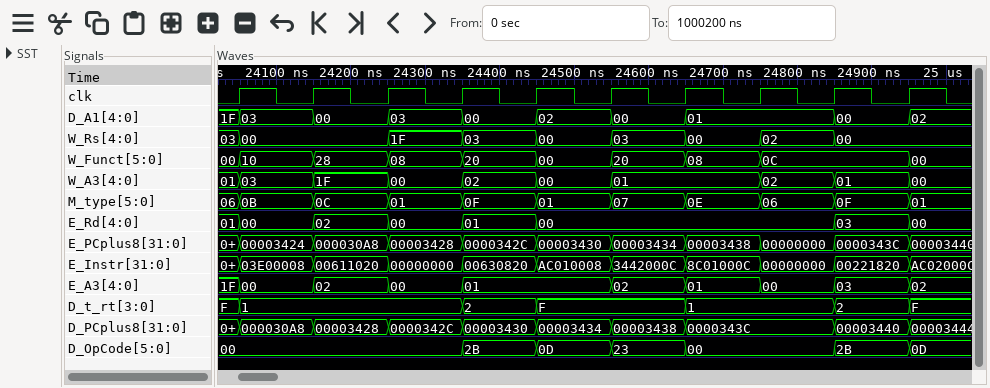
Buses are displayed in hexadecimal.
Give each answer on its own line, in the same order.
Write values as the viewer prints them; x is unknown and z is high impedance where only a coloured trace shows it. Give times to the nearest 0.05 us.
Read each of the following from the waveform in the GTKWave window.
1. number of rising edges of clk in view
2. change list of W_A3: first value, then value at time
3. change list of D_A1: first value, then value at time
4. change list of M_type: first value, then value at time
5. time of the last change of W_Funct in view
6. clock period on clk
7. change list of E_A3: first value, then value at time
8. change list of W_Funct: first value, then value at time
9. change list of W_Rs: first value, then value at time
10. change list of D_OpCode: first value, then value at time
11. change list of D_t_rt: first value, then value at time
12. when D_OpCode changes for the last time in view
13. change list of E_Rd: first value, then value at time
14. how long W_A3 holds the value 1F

10
01, 03 at 24.05 us, 1F at 24.15 us, 00 at 24.25 us, 02 at 24.35 us, 00 at 24.45 us, 01 at 24.55 us, 02 at 24.75 us, 01 at 24.85 us, 00 at 24.95 us
1F, 03 at 24.05 us, 00 at 24.15 us, 03 at 24.25 us, 00 at 24.35 us, 02 at 24.45 us, 00 at 24.55 us, 01 at 24.65 us, 00 at 24.85 us, 02 at 24.95 us
06, 0B at 24.05 us, 0C at 24.15 us, 01 at 24.25 us, 0F at 24.35 us, 01 at 24.45 us, 07 at 24.55 us, 0E at 24.65 us, 06 at 24.75 us, 0F at 24.85 us, 01 at 24.95 us
24.95 us
0.1 us
1F, 00 at 24.05 us, 02 at 24.15 us, 00 at 24.25 us, 01 at 24.35 us, 02 at 24.55 us, 01 at 24.65 us, 00 at 24.75 us, 03 at 24.85 us, 02 at 24.95 us
00, 10 at 24.05 us, 28 at 24.15 us, 08 at 24.25 us, 20 at 24.35 us, 00 at 24.45 us, 20 at 24.55 us, 08 at 24.65 us, 0C at 24.75 us, 00 at 24.95 us
03, 00 at 24.05 us, 1F at 24.25 us, 03 at 24.35 us, 00 at 24.45 us, 03 at 24.55 us, 00 at 24.65 us, 02 at 24.75 us, 00 at 24.85 us
00, 2B at 24.35 us, 0D at 24.45 us, 23 at 24.55 us, 00 at 24.65 us, 2B at 24.85 us, 0D at 24.95 us
F, 1 at 24.05 us, 2 at 24.35 us, F at 24.45 us, 1 at 24.65 us, 2 at 24.85 us, F at 24.95 us
24.95 us
01, 00 at 24.05 us, 02 at 24.15 us, 00 at 24.25 us, 01 at 24.35 us, 00 at 24.45 us, 03 at 24.85 us, 00 at 24.95 us
0.1 us
